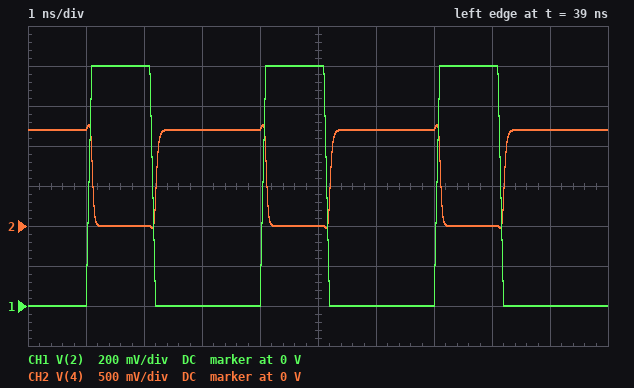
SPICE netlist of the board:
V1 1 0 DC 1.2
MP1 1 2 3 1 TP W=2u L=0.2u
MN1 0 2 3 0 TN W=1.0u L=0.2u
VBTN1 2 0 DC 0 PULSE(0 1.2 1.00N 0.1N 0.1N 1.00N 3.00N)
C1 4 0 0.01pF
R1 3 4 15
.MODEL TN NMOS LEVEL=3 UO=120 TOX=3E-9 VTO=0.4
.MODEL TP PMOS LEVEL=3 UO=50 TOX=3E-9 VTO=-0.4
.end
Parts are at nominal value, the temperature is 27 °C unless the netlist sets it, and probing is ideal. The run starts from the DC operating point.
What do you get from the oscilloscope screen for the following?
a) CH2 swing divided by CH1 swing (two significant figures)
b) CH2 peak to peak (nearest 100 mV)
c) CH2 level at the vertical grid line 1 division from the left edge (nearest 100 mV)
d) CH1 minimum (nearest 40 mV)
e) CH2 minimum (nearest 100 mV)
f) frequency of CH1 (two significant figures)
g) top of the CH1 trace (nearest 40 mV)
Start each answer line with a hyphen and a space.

- 1.1
- 1.3 V
- 1.2 V
- 0 V
- 0 V
- 330 MHz
- 1.20 V
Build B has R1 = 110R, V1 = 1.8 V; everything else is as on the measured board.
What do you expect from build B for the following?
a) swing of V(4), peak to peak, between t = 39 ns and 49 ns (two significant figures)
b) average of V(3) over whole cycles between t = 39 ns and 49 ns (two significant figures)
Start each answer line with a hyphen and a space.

- 1.8 V
- 1.2 V
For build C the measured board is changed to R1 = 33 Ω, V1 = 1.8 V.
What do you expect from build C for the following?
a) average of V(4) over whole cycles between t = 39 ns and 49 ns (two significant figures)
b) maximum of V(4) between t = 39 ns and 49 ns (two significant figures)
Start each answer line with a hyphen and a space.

- 1.2 V
- 1.8 V
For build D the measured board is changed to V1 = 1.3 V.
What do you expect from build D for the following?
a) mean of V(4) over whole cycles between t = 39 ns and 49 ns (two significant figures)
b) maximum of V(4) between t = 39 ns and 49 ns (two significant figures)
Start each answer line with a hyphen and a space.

- 830 mV
- 1.4 V
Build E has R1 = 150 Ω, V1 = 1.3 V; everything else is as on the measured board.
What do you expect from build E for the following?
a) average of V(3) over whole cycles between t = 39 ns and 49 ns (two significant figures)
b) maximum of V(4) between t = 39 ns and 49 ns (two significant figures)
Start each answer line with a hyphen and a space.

- 830 mV
- 1.4 V
